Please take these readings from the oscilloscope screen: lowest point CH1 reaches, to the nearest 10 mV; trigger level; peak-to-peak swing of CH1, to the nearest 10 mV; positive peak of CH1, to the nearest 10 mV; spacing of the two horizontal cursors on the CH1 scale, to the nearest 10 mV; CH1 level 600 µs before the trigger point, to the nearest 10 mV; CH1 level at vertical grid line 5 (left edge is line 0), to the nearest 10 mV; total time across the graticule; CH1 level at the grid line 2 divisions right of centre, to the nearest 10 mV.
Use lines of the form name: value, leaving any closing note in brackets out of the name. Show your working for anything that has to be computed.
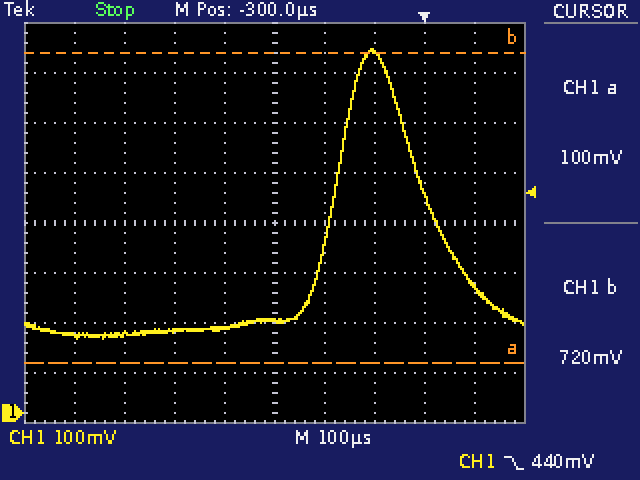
lowest point CH1 reaches, to the nearest 10 mV: 150 mV
trigger level: 440 mV
peak-to-peak swing of CH1, to the nearest 10 mV: 730 mV − (150 mV) = 580 mV
positive peak of CH1, to the nearest 10 mV: 730 mV
spacing of the two horizontal cursors on the CH1 scale, to the nearest 10 mV: 620 mV
CH1 level 600 µs before the trigger point, to the nearest 10 mV: 160 mV
CH1 level at vertical grid line 5 (left edge is line 0), to the nearest 10 mV: 180 mV
total time across the graticule: 1 ms
CH1 level at the grid line 2 divisions right of centre, to the nearest 10 mV: 720 mV
